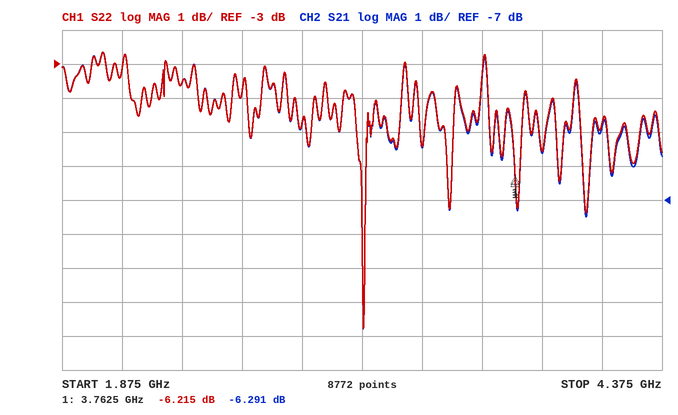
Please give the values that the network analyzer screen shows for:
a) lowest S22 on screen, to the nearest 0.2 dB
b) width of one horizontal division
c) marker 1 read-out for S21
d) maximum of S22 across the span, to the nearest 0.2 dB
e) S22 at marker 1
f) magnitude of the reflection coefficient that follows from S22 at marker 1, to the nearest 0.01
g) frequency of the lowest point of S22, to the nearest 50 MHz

-10.8 dB
250 MHz
-6.291 dB
-2.6 dB
-6.215 dB
0.49
3.15 GHz
